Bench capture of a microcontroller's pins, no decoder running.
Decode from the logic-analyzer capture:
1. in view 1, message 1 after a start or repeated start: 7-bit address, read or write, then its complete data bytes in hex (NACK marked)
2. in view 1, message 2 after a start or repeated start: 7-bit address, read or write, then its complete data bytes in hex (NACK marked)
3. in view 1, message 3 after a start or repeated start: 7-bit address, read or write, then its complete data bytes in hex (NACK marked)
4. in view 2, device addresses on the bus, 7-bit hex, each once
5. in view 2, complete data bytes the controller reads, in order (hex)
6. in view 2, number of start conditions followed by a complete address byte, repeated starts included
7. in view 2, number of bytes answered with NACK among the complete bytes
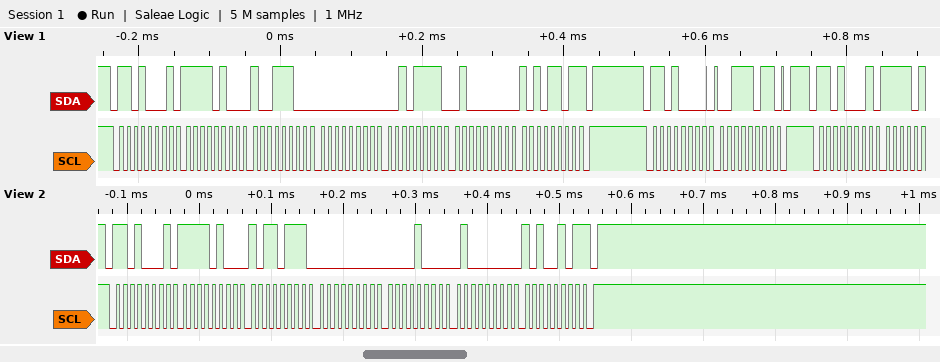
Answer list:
0x68 read: F4 9C 00 2F 40 AD NACK
0x68 write: 3B
0x68 read
0x68
F4 B7 00 08 40 A5
1
1
